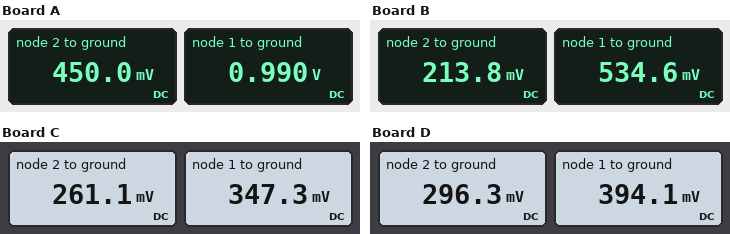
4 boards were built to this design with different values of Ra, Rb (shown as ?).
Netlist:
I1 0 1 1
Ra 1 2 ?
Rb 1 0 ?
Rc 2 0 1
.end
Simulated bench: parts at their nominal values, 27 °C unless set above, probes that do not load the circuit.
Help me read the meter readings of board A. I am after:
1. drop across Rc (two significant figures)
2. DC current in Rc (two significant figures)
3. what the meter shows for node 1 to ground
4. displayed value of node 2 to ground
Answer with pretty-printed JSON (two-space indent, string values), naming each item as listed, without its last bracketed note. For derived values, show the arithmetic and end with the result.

{
  "drop across Rc": "450 mV = 450 mV",
  "DC current in Rc": "(450 mV) / 1 Ω = 450 mA",
  "what the meter shows for node 1 to ground": "0.990 V",
  "displayed value of node 2 to ground": "450.0 mV"
}
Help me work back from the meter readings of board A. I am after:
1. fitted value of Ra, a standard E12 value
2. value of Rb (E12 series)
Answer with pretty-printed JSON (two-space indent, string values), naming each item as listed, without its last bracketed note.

{
  "fitted value of Ra, a standard E12 value": "1.2 Ω",
  "value of Rb": "1.8 Ω"
}
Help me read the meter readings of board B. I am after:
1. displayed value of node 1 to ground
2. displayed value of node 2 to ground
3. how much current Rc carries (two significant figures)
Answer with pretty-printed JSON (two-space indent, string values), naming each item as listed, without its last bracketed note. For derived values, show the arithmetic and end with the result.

{
  "displayed value of node 1 to ground": "534.6 mV",
  "displayed value of node 2 to ground": "213.8 mV",
  "how much current Rc carries": "(213.8 mV) / 1 Ω = 210 mA"
}
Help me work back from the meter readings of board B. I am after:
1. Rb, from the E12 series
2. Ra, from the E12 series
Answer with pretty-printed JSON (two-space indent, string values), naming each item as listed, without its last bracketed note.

{
  "Rb, from the E12 series": "0.68 Ω",
  "Ra, from the E12 series": "1.5 Ω"
}
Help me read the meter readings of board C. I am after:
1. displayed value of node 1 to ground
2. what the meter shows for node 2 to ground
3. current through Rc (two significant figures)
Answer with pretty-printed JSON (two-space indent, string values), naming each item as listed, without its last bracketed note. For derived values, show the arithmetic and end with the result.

{
  "displayed value of node 1 to ground": "347.3 mV",
  "what the meter shows for node 2 to ground": "261.1 mV",
  "current through Rc": "(261.1 mV) / 1 Ω = 260 mA"
}
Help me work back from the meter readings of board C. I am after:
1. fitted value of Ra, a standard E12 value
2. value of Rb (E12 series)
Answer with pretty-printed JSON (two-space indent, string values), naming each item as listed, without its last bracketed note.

{
  "fitted value of Ra, a standard E12 value": "0.33 Ω",
  "value of Rb": "0.47 Ω"
}
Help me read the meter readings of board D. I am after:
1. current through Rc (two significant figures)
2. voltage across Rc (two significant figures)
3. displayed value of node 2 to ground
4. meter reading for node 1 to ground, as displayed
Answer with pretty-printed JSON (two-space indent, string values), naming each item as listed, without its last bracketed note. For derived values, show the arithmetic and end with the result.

{
  "current through Rc": "(296.3 mV) / 1 Ω = 300 mA",
  "voltage across Rc": "296.3 mV = 300 mV",
  "displayed value of node 2 to ground": "296.3 mV",
  "meter reading for node 1 to ground, as displayed": "394.1 mV"
}
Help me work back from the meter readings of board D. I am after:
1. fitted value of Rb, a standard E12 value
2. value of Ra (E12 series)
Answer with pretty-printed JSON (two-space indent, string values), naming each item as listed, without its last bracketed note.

{
  "fitted value of Rb, a standard E12 value": "0.56 Ω",
  "value of Ra": "0.33 Ω"
}
